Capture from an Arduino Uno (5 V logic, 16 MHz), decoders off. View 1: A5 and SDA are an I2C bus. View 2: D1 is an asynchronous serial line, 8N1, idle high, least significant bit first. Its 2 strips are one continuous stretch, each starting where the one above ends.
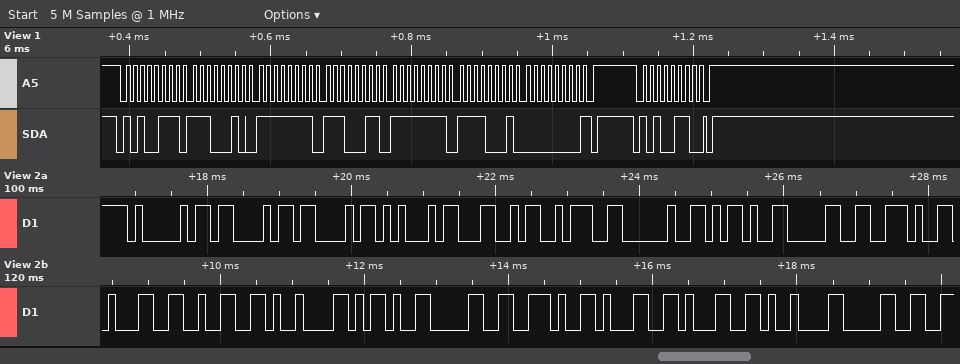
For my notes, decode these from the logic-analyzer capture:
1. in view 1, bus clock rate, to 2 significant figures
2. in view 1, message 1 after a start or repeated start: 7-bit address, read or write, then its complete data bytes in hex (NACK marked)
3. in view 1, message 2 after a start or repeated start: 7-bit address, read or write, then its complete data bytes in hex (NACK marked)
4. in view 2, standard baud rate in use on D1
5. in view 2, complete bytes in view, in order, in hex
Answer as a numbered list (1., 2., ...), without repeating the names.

1. 100 kHz
2. 0x53 read: E2 FF E3 FF F1 00 NACK
3. 0x53 write
4. 9600 baud
5. 41 43 43 45 4C 3A 20 2D 30 2E 31 32 09 2D 30 2E 31 31 09 30
